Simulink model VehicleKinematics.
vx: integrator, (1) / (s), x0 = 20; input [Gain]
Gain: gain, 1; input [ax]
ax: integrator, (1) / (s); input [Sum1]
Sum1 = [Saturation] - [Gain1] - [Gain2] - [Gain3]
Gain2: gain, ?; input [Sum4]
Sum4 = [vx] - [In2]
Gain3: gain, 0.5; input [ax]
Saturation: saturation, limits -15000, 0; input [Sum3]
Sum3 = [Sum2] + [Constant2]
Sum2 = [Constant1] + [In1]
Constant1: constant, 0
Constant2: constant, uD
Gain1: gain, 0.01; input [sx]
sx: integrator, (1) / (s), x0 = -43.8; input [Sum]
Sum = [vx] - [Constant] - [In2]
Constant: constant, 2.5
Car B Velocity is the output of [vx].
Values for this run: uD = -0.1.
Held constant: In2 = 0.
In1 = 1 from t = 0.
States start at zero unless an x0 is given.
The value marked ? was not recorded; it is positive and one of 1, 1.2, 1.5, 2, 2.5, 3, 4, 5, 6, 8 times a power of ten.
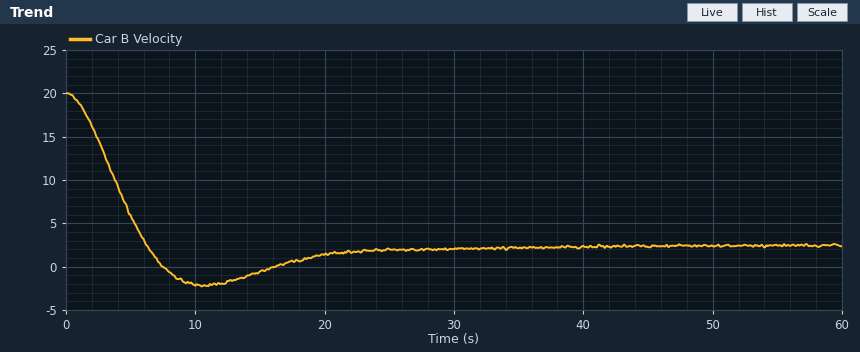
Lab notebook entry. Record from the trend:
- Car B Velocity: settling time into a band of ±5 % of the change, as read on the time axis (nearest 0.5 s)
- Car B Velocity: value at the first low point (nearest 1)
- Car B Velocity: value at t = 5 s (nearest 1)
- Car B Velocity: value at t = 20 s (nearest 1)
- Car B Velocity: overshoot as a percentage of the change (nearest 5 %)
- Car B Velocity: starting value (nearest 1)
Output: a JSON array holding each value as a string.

["21.5 s", "-2", "6", "1", "25 %", "20"]
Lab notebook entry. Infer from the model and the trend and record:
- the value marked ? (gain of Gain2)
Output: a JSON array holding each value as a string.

["0.15"]
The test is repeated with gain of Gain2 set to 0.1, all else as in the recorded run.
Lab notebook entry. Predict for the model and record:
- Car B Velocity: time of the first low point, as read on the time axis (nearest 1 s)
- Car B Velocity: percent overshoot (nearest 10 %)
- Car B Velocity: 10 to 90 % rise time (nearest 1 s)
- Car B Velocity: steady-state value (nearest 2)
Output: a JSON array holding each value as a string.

["15 s", "30 %", "6 s", "2"]
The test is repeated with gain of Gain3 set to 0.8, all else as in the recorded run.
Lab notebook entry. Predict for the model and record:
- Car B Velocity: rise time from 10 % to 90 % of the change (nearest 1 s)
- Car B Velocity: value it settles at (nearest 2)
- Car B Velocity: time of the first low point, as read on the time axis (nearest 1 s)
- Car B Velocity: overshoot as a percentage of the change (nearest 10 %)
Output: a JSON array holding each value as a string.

["6 s", "2", "17 s", "20 %"]
